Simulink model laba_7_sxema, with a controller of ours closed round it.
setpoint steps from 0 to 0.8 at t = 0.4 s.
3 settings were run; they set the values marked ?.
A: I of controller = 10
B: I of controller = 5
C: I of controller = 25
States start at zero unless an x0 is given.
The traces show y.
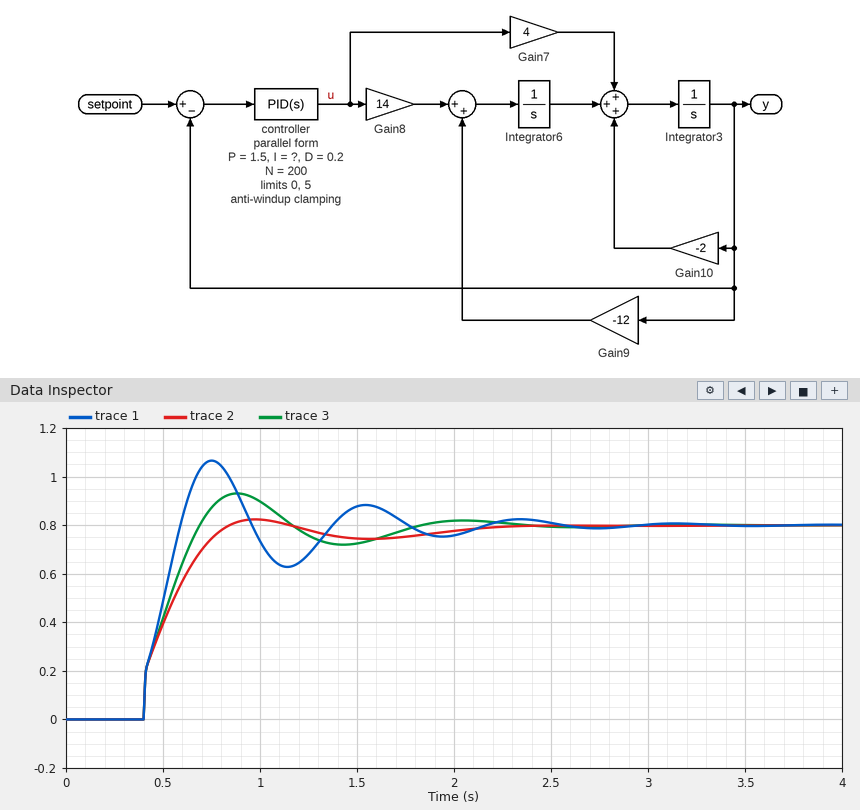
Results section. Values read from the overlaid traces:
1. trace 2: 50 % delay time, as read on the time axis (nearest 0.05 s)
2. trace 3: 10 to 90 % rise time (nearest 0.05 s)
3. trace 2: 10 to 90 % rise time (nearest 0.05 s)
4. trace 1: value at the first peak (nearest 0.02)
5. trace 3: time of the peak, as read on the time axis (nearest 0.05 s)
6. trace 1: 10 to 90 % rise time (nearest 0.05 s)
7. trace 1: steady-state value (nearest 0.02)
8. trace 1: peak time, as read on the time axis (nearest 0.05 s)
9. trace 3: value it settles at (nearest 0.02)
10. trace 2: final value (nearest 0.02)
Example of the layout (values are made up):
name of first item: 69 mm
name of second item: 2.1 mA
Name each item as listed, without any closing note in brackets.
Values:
trace 2: 50 % delay time, as read on the time axis: 0.50 s
trace 3: 10 to 90 % rise time: 0.25 s
trace 2: 10 to 90 % rise time: 0.30 s
trace 1: value at the first peak: 1.06
trace 3: time of the peak, as read on the time axis: 0.90 s
trace 1: 10 to 90 % rise time: 0.15 s
trace 1: steady-state value: 0.80
trace 1: peak time, as read on the time axis: 0.75 s
trace 3: value it settles at: 0.80
trace 2: final value: 0.80
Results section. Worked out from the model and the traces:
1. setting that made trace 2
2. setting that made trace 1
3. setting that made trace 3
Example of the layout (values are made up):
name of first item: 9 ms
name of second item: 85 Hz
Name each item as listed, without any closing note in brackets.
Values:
setting that made trace 2: B
setting that made trace 1: C
setting that made trace 3: A
